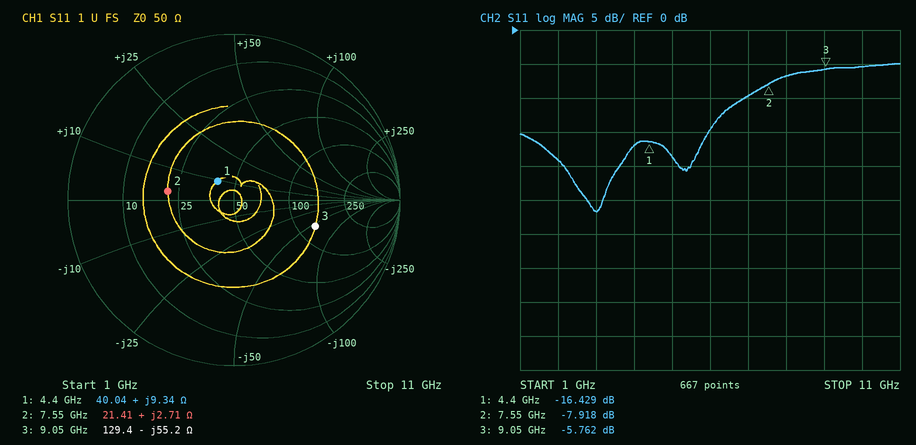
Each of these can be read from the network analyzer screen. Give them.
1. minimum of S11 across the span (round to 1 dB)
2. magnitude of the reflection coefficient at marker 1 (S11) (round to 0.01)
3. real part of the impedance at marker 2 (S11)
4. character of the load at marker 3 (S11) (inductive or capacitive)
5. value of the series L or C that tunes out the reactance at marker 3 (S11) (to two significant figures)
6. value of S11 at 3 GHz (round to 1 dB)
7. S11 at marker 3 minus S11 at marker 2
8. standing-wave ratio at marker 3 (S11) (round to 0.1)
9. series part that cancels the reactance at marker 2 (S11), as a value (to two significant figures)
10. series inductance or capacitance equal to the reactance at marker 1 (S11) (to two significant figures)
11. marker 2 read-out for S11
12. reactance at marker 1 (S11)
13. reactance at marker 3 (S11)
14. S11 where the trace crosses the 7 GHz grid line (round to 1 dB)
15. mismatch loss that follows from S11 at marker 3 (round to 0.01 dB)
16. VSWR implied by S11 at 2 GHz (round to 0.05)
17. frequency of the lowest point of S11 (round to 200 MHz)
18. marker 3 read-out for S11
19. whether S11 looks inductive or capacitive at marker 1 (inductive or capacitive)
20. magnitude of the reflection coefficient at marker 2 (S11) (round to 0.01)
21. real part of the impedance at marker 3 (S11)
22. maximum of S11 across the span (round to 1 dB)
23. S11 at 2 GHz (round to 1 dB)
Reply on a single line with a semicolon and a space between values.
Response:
-27 dB; 0.15; 21.41 Ω; capacitive; 970 pH; -27 dB; 2.156 dB; 3.1; 7.8 pF; 340 pH; -7.918 dB; +9.34 Ω; -55.2 Ω; -10 dB; 1.34 dB; 1.25; 3.0 GHz; -5.762 dB; inductive; 0.40; 129.4 Ω; -5 dB; -19 dB
